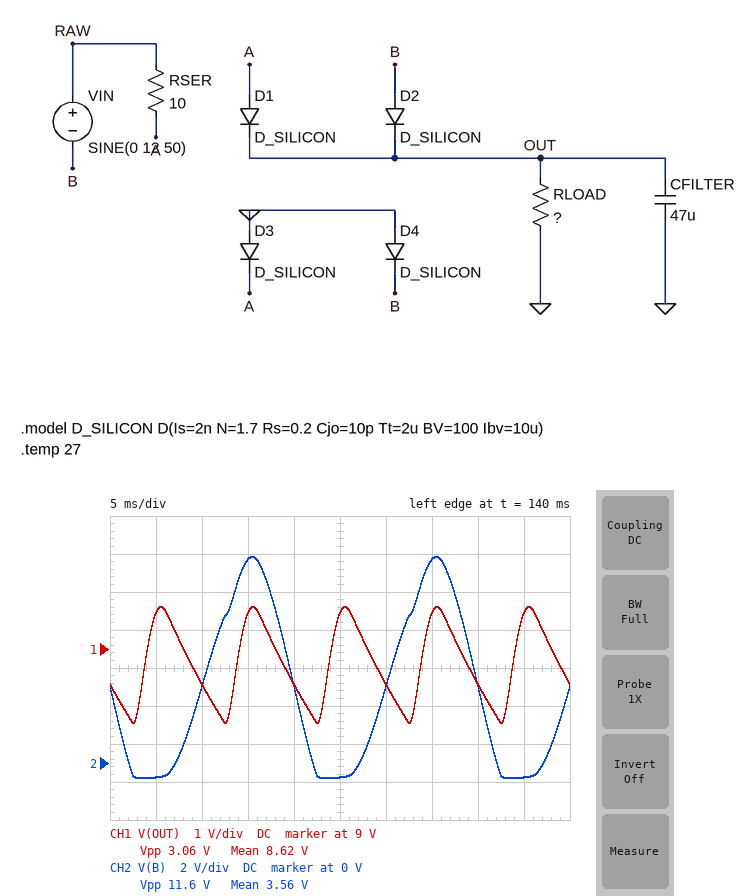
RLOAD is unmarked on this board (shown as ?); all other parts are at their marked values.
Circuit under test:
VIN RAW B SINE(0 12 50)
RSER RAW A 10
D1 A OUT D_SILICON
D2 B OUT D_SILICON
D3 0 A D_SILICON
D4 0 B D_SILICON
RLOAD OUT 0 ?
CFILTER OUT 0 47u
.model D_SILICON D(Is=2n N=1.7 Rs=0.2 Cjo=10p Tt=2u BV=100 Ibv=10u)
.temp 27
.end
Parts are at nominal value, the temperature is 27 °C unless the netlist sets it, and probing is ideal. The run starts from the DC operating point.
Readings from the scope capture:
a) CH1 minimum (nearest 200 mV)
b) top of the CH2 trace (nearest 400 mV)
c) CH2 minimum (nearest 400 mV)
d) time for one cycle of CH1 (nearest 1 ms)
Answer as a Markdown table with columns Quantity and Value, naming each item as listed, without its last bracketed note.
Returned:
| Quantity | Value |
|---|---|
| CH1 minimum | 7.0 V |
| top of the CH2 trace | 10.8 V |
| CH2 minimum | -800 mV |
| time for one cycle of CH1 | 10 ms |
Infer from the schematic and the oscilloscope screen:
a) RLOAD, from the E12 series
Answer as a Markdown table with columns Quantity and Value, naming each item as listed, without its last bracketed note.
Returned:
| Quantity | Value |
|---|---|
| RLOAD, from the E12 series | 390 Ω |
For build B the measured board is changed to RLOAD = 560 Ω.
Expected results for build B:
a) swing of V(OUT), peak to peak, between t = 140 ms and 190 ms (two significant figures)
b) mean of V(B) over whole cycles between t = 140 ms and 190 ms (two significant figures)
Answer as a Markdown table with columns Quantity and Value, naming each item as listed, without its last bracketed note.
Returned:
| Quantity | Value |
|---|---|
| swing of V(OUT), peak to peak, between t = 140 ms and 190 ms | 2.4 V |
| mean of V(B) over whole cycles between t = 140 ms and 190 ms | 4.5 V |
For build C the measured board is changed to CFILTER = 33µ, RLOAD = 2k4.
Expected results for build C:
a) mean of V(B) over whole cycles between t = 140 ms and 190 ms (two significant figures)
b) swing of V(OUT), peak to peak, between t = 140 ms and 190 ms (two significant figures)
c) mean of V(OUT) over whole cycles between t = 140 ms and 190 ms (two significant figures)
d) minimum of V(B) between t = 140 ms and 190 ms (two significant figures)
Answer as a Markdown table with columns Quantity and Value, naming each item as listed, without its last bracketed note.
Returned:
| Quantity | Value |
|---|---|
| mean of V(B) over whole cycles between t = 140 ms and 190 ms | 5.0 V |
| swing of V(OUT), peak to peak, between t = 140 ms and 190 ms | 990 mV |
| mean of V(OUT) over whole cycles between t = 140 ms and 190 ms | 10 V |
| minimum of V(B) between t = 140 ms and 190 ms | -740 mV |
